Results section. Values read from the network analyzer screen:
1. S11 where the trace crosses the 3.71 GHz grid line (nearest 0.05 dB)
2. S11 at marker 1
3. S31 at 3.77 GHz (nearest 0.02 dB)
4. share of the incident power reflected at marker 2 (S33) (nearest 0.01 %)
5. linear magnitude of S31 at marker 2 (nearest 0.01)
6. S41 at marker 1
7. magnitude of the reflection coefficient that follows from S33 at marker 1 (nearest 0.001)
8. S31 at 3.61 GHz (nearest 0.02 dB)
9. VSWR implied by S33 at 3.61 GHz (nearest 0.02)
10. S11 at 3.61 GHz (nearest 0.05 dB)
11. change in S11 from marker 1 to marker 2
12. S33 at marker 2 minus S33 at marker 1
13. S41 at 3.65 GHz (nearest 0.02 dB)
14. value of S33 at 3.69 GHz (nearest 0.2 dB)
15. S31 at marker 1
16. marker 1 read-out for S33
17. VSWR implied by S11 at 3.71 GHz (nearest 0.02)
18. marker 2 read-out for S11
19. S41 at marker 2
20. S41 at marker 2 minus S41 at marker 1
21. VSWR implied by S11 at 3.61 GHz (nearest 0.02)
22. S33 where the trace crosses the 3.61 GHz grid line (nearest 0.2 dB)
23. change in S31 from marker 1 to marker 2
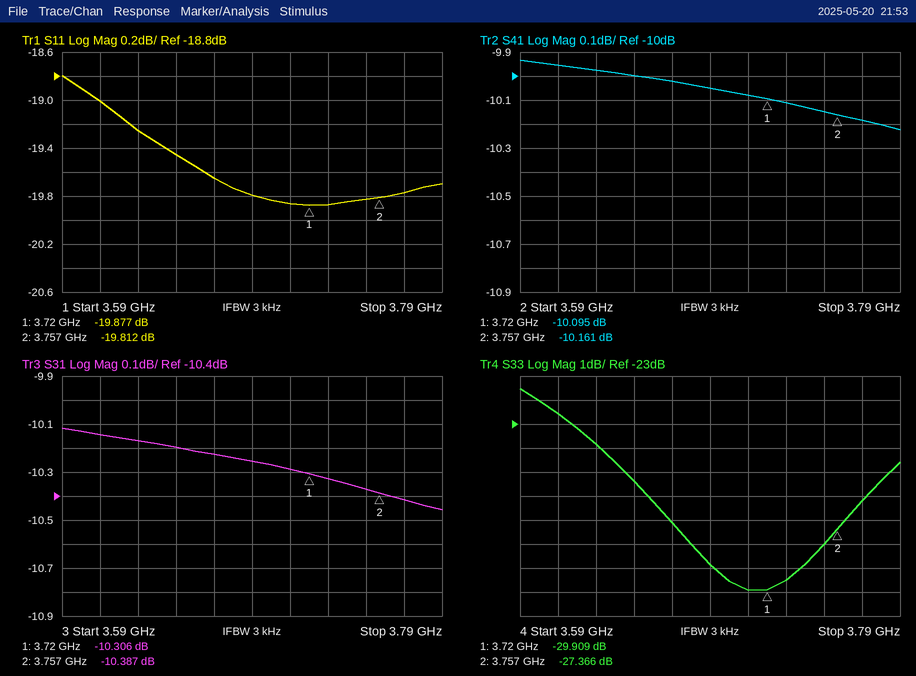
-19.85 dB
-19.877 dB
-10.42 dB
0.18 %
0.30
-10.095 dB
0.032
-10.14 dB
1.16
-19.00 dB
0.065 dB
2.543 dB
-10.00 dB
-28.8 dB
-10.306 dB
-29.909 dB
1.22
-19.812 dB
-10.161 dB
-0.066 dB
1.26
-22.6 dB
-0.081 dB
